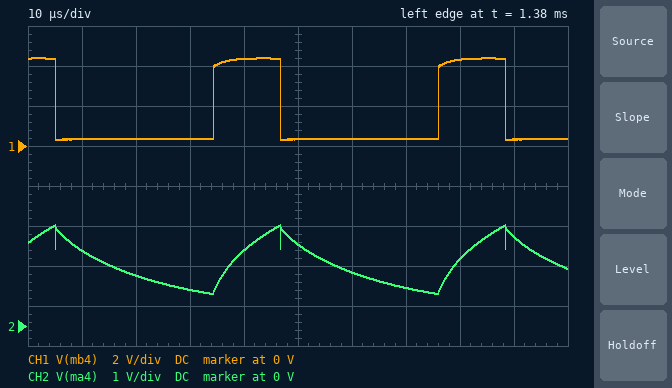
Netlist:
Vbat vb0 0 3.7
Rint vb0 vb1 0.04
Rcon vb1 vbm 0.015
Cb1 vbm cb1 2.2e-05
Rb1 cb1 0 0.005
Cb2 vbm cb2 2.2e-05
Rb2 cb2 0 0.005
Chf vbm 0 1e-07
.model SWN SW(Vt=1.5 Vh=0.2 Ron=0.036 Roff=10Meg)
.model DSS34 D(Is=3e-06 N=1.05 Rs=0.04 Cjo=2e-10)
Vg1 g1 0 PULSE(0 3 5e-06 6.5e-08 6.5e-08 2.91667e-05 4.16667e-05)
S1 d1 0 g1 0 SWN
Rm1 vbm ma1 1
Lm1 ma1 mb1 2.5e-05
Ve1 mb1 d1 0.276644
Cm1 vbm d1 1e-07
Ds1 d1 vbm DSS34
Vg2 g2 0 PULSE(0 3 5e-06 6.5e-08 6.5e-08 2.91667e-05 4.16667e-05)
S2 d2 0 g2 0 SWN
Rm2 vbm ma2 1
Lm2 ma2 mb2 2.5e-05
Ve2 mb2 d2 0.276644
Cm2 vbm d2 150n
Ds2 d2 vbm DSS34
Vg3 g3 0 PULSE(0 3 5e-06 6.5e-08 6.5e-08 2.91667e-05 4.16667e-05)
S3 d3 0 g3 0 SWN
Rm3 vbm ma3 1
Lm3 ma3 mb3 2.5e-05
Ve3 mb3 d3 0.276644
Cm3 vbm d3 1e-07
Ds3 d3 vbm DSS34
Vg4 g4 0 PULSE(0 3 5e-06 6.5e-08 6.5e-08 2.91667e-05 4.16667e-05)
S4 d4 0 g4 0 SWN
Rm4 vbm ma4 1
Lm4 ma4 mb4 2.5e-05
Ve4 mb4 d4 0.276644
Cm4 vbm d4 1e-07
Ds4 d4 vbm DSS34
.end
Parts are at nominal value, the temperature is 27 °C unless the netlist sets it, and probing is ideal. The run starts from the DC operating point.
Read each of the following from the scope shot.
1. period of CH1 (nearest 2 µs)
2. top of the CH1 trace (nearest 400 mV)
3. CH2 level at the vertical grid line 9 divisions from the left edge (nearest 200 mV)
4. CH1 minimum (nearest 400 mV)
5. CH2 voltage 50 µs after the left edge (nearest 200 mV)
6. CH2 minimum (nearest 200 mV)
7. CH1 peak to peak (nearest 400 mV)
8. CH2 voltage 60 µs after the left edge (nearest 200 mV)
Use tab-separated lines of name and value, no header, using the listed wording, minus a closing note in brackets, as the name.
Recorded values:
period of CH1	42 µs
top of the CH1 trace	4.4 V
CH2 level at the vertical grid line 9 divisions from the left edge	2.2 V
CH1 minimum	400 mV
CH2 voltage 50 µs after the left edge	2.0 V
CH2 minimum	800 mV
CH1 peak to peak	4.0 V
CH2 voltage 60 µs after the left edge	1.4 V
